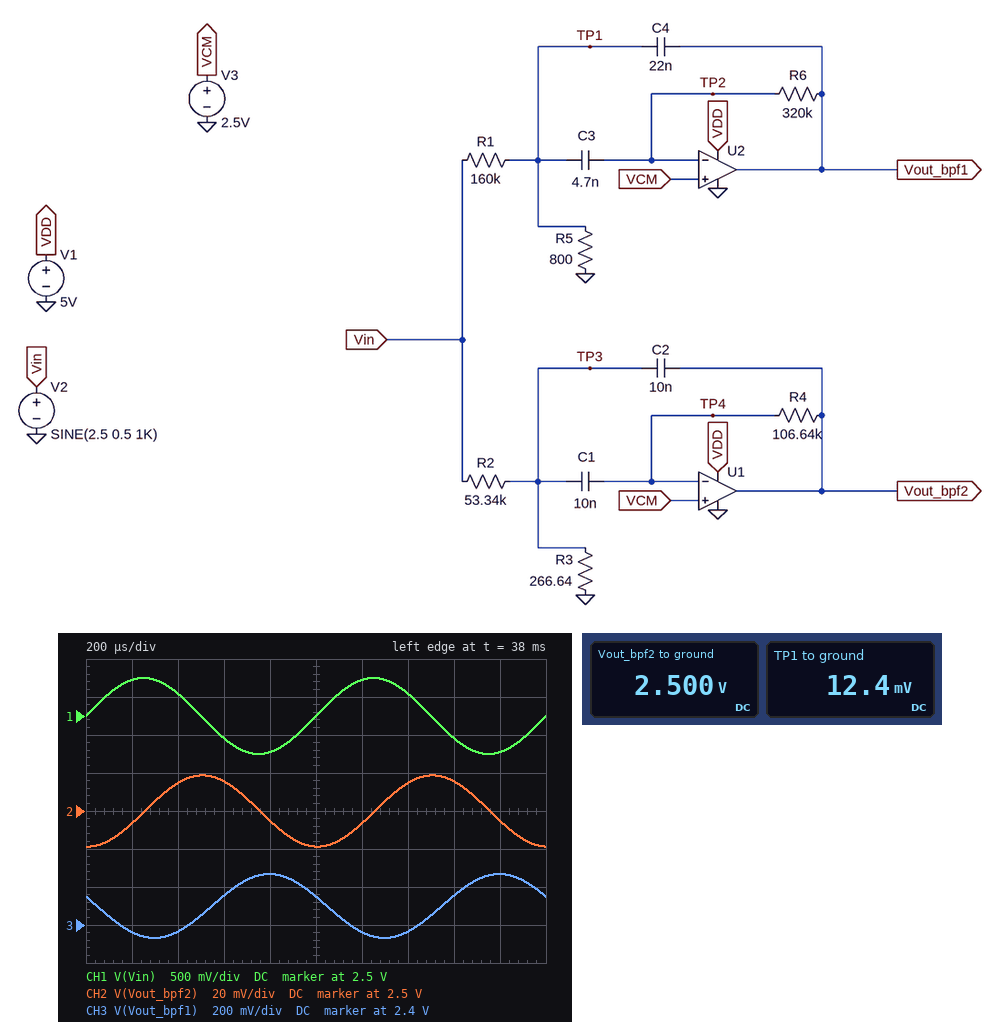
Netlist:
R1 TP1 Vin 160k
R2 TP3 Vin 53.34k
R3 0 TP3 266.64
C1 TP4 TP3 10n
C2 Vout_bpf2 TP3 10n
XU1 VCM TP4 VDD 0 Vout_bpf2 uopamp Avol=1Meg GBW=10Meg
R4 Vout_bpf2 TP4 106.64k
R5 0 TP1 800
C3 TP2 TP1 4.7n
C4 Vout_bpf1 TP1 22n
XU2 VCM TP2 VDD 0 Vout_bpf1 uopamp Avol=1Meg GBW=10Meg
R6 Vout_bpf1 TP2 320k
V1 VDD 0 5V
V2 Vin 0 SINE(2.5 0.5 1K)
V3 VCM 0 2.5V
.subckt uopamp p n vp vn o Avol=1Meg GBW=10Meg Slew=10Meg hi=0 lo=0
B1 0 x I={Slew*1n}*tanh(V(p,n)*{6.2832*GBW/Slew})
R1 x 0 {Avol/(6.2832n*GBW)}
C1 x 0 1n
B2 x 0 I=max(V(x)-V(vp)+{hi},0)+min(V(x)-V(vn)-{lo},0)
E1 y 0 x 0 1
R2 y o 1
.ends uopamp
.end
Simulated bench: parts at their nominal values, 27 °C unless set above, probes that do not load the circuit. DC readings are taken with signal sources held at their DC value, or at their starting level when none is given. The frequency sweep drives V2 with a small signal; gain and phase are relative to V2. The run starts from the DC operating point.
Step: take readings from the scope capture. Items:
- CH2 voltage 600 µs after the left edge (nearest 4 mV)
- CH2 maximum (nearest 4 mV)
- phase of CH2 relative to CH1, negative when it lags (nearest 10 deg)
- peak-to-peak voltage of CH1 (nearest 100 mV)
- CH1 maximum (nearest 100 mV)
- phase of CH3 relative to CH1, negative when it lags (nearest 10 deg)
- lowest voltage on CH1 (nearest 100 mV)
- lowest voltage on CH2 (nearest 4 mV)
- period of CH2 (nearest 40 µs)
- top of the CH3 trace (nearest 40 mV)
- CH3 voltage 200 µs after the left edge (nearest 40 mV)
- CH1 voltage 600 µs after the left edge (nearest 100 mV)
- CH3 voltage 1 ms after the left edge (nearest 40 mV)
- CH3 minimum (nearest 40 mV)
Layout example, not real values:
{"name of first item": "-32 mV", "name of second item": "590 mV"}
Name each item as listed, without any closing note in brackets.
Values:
{"CH2 voltage 600 µs after the left edge": "2.516 V", "CH2 maximum": "2.520 V", "phase of CH2 relative to CH1, negative when it lags": "-90 deg", "peak-to-peak voltage of CH1": "1.0 V", "CH1 maximum": "3.0 V", "phase of CH3 relative to CH1, negative when it lags": "160 deg", "lowest voltage on CH1": "2.0 V", "lowest voltage on CH2": "2.480 V", "period of CH2": "1.00 ms", "top of the CH3 trace": "2.68 V", "CH3 voltage 200 µs after the left edge": "2.36 V", "CH1 voltage 600 µs after the left edge": "2.2 V", "CH3 voltage 1 ms after the left edge": "2.56 V", "CH3 minimum": "2.32 V"}
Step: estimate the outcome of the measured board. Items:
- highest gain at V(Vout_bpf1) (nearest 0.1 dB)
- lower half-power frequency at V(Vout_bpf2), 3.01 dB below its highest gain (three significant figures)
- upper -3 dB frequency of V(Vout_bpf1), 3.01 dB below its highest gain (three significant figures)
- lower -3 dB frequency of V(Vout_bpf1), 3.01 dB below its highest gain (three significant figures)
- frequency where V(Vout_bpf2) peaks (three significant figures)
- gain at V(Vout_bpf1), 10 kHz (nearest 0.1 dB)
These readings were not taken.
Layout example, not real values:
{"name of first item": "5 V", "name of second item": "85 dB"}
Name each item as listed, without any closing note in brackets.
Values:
{"highest gain at V(Vout_bpf1)": "-9.1 dB", "lower half-power frequency at V(Vout_bpf2), 3.01 dB below its highest gain": "2.84 kHz", "upper -3 dB frequency of V(Vout_bpf1), 3.01 dB below its highest gain": "1.05 kHz", "lower -3 dB frequency of V(Vout_bpf1), 3.01 dB below its highest gain": "918 Hz", "frequency where V(Vout_bpf2) peaks": "2.98 kHz", "gain at V(Vout_bpf1), 10 kHz": "-46.8 dB"}
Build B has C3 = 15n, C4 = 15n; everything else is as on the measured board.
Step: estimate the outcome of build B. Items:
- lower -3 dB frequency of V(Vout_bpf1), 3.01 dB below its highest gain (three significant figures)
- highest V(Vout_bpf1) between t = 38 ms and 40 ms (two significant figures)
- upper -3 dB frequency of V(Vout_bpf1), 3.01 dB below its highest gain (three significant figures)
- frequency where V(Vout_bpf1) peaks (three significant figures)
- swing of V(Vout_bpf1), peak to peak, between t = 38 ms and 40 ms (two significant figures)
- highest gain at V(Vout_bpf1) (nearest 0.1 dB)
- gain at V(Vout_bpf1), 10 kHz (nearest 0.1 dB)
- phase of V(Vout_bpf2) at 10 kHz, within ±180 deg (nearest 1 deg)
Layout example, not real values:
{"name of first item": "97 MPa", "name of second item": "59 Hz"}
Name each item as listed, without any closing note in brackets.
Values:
{"lower -3 dB frequency of V(Vout_bpf1), 3.01 dB below its highest gain": "632 Hz", "highest V(Vout_bpf1) between t = 38 ms and 40 ms": "2.6 V", "upper -3 dB frequency of V(Vout_bpf1), 3.01 dB below its highest gain": "698 Hz", "frequency where V(Vout_bpf1) peaks": "664 Hz", "swing of V(Vout_bpf1), peak to peak, between t = 38 ms and 40 ms": "120 mV", "highest gain at V(Vout_bpf1)": "0 dB", "gain at V(Vout_bpf1), 10 kHz": "-43.5 dB", "phase of V(Vout_bpf2) at 10 kHz, within ±180 deg": "92 deg"}
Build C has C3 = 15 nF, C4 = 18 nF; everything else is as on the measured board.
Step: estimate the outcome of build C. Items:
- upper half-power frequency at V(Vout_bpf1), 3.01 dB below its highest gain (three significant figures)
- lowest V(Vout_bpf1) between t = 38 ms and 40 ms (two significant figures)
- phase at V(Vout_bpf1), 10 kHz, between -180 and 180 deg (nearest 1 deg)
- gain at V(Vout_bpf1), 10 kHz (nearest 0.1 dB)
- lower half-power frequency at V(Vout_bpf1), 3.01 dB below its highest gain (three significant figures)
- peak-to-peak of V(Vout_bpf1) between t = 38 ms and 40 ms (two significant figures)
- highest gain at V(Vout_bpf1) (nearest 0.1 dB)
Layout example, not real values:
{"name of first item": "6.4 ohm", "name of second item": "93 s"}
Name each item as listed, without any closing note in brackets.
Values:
{"upper half-power frequency at V(Vout_bpf1), 3.01 dB below its highest gain": "638 Hz", "lowest V(Vout_bpf1) between t = 38 ms and 40 ms": "2.5 V", "phase at V(Vout_bpf1), 10 kHz, between -180 and 180 deg": "90 deg", "gain at V(Vout_bpf1), 10 kHz": "-45.1 dB", "lower half-power frequency at V(Vout_bpf1), 3.01 dB below its highest gain": "577 Hz", "peak-to-peak of V(Vout_bpf1) between t = 38 ms and 40 ms": "87 mV", "highest gain at V(Vout_bpf1)": "-0.8 dB"}
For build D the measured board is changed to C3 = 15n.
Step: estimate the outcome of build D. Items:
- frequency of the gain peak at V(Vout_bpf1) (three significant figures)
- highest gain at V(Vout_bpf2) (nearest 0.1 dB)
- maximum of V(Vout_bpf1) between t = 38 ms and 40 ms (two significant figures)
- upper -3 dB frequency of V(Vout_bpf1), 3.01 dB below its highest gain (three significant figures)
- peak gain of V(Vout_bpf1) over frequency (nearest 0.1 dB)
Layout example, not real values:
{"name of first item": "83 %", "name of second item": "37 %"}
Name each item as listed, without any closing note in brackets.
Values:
{"frequency of the gain peak at V(Vout_bpf1)": "549 Hz", "highest gain at V(Vout_bpf2)": "0 dB", "maximum of V(Vout_bpf1) between t = 38 ms and 40 ms": "2.5 V", "upper -3 dB frequency of V(Vout_bpf1), 3.01 dB below its highest gain": "577 Hz", "peak gain of V(Vout_bpf1) over frequency": "-1.8 dB"}
